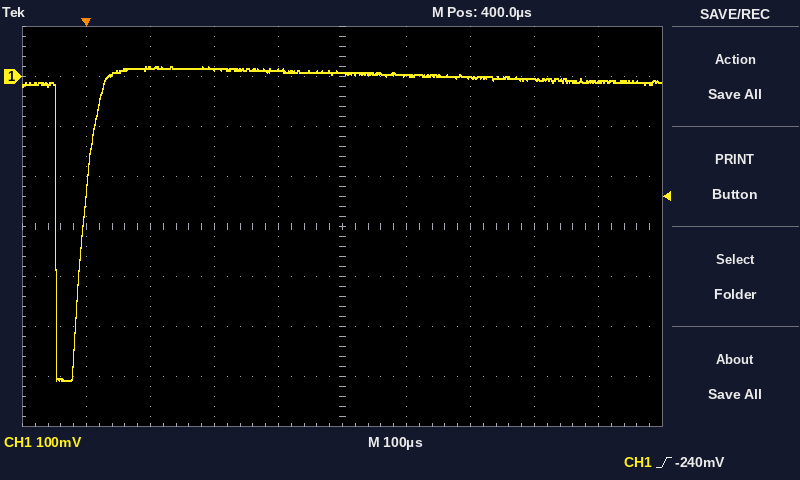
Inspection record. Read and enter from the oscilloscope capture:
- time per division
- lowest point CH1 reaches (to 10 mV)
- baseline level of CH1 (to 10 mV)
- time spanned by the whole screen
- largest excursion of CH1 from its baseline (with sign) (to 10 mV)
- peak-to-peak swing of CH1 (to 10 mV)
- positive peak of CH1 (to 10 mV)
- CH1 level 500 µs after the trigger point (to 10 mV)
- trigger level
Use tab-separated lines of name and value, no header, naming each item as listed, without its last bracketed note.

time per division	100 µs
lowest point CH1 reaches	-610 mV
baseline level of CH1	0 mV
time spanned by the whole screen	1 ms
largest excursion of CH1 from its baseline (with sign)	-610 mV
peak-to-peak swing of CH1	630 mV
positive peak of CH1	20 mV
CH1 level 500 µs after the trigger point	0 mV
trigger level	-240 mV
